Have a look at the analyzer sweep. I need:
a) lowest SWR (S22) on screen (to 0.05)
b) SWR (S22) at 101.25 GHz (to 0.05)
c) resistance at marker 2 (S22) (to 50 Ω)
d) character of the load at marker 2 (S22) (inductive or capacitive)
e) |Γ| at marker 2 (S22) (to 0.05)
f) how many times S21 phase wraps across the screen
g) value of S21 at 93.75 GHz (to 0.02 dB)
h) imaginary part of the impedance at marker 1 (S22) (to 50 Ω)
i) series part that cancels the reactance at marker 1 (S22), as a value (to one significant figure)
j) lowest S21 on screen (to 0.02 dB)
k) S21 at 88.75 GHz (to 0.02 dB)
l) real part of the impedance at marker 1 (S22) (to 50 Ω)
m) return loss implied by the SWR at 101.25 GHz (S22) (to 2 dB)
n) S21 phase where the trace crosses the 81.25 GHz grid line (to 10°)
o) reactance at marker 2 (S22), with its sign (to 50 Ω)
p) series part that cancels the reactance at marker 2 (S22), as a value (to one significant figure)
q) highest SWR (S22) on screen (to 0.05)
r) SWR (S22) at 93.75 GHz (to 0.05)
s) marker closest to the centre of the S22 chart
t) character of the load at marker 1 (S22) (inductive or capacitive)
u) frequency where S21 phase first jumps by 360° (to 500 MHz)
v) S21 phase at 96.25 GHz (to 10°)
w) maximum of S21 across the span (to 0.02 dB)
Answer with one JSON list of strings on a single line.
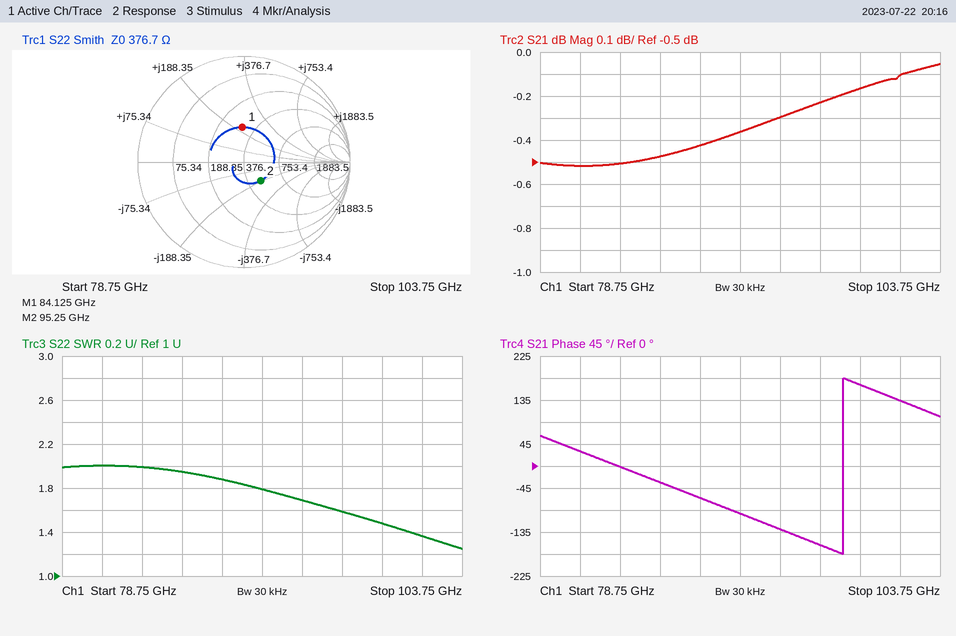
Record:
["1.25", "1.35", "500 Ω", "capacitive", "0.25", "1", "-0.30 dB", "+200 Ω", "9 fF", "-0.52 dB", "-0.42 dB", "300 Ω", "16 dB", "30°", "-200 Ω", "300 pH", "2.00", "1.70", "marker 2", "inductive", "97.5 GHz", "-160°", "-0.06 dB"]
